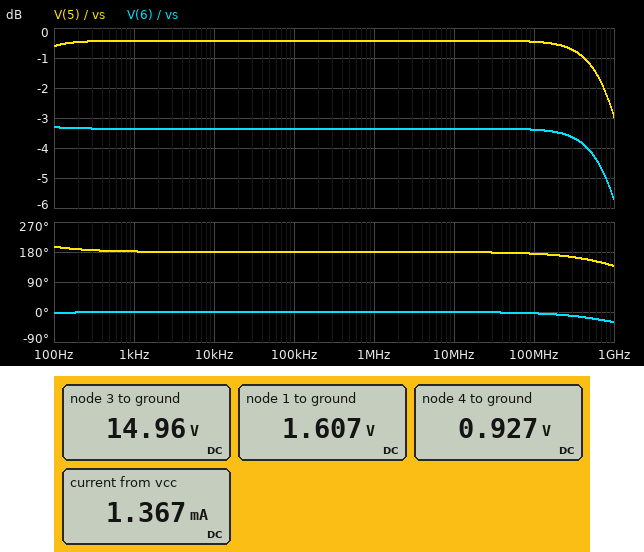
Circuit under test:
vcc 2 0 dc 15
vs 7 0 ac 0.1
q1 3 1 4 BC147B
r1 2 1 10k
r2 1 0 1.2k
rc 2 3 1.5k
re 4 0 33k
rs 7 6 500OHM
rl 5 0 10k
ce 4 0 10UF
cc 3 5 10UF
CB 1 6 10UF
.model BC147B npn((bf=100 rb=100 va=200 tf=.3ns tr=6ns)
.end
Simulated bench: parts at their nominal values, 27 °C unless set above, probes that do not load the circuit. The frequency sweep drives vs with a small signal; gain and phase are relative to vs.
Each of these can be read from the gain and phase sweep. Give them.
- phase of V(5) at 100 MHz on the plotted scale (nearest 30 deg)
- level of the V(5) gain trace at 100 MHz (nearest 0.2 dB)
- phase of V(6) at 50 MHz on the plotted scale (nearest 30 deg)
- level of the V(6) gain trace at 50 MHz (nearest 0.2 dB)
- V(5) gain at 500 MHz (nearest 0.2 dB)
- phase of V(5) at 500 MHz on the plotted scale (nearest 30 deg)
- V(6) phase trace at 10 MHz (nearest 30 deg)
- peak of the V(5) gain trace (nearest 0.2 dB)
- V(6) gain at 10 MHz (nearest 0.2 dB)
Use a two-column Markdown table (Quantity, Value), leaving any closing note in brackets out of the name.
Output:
| Quantity | Value |
|---|---|
| phase of V(5) at 100 MHz on the plotted scale | 180 deg |
| level of the V(5) gain trace at 100 MHz | -0.4 dB |
| phase of V(6) at 50 MHz on the plotted scale | 0 deg |
| level of the V(6) gain trace at 50 MHz | -3.4 dB |
| V(5) gain at 500 MHz | -1.2 dB |
| phase of V(5) at 500 MHz on the plotted scale | 150 deg |
| V(6) phase trace at 10 MHz | 0 deg |
| peak of the V(5) gain trace | -0.4 dB |
| V(6) gain at 10 MHz | -3.4 dB |
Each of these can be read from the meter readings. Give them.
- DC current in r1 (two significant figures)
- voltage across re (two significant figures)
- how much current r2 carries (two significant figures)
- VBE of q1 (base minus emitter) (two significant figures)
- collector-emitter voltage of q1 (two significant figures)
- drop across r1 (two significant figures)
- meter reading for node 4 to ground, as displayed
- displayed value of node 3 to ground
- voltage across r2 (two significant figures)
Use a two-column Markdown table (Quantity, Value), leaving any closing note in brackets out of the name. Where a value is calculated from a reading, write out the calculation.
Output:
| Quantity | Value |
|---|---|
| DC current in r1 | (15 V - 1.607 V) / 10 kΩ = 1.3 mA |
| voltage across re | 927 mV = 930 mV |
| how much current r2 carries | (1.607 V) / 1.2 kΩ = 1.3 mA |
| VBE of q1 (base minus emitter) | 1.607 V - 927 mV = 680 mV |
| collector-emitter voltage of q1 | 14.96 V - 927 mV = 14 V |
| drop across r1 | 15 V - 1.607 V = 13 V |
| meter reading for node 4 to ground, as displayed | 0.927 V |
| displayed value of node 3 to ground | 14.96 V |
| voltage across r2 | 1.607 V = 1.6 V |
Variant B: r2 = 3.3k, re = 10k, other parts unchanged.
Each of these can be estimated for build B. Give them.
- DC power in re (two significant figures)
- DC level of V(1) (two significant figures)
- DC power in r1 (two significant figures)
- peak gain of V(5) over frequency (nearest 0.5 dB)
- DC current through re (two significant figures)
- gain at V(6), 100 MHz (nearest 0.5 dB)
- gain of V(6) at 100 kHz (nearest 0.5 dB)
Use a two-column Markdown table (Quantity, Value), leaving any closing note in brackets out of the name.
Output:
| Quantity | Value |
|---|---|
| DC power in re | 880 µW |
| DC level of V(1) | 3.7 V |
| DC power in r1 | 13 mW |
| peak gain of V(5) over frequency | 21.5 dB |
| DC current through re | 300 µA |
| gain at V(6), 100 MHz | -5.0 dB |
| gain of V(6) at 100 kHz | -2.0 dB |
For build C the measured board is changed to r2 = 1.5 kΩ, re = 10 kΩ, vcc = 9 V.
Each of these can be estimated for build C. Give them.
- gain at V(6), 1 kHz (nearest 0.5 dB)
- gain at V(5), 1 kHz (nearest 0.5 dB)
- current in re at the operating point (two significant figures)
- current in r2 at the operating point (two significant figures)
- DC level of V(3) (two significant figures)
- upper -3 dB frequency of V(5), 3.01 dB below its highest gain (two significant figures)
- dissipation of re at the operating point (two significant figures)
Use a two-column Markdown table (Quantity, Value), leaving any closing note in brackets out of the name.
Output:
| Quantity | Value |
|---|---|
| gain at V(6), 1 kHz | -3.0 dB |
| gain at V(5), 1 kHz | 4.5 dB |
| current in re at the operating point | 48 µA |
| current in r2 at the operating point | 780 µA |
| DC level of V(3) | 8.9 V |
| upper -3 dB frequency of V(5), 3.01 dB below its highest gain | 630 MHz |
| dissipation of re at the operating point | 23 µW |
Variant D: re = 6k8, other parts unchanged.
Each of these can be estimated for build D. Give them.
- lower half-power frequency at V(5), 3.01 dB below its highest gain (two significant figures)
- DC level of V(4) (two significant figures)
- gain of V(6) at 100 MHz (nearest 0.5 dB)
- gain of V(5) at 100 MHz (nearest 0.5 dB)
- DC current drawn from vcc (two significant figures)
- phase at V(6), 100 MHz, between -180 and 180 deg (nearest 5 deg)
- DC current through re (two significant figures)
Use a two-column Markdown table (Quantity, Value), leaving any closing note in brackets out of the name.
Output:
| Quantity | Value |
|---|---|
| lower half-power frequency at V(5), 3.01 dB below its highest gain | 82 Hz |
| DC level of V(4) | 890 mV |
| gain of V(6) at 100 MHz | -4.0 dB |
| gain of V(5) at 100 MHz | 12.0 dB |
| DC current drawn from vcc | 1.5 mA |
| phase at V(6), 100 MHz, between -180 and 180 deg | -15 deg |
| DC current through re | 130 µA |
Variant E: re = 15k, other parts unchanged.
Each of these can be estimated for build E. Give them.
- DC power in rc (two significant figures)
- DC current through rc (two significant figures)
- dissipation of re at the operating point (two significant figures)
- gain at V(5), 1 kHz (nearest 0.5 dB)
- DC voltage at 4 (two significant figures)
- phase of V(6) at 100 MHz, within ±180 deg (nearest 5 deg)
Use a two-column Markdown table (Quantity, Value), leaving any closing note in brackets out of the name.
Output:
| Quantity | Value |
|---|---|
| DC power in rc | 5.4 µW |
| DC current through rc | 60 µA |
| dissipation of re at the operating point | 55 µW |
| gain at V(5), 1 kHz | 6.0 dB |
| DC voltage at 4 | 910 mV |
| phase of V(6) at 100 MHz, within ±180 deg | -10 deg |
